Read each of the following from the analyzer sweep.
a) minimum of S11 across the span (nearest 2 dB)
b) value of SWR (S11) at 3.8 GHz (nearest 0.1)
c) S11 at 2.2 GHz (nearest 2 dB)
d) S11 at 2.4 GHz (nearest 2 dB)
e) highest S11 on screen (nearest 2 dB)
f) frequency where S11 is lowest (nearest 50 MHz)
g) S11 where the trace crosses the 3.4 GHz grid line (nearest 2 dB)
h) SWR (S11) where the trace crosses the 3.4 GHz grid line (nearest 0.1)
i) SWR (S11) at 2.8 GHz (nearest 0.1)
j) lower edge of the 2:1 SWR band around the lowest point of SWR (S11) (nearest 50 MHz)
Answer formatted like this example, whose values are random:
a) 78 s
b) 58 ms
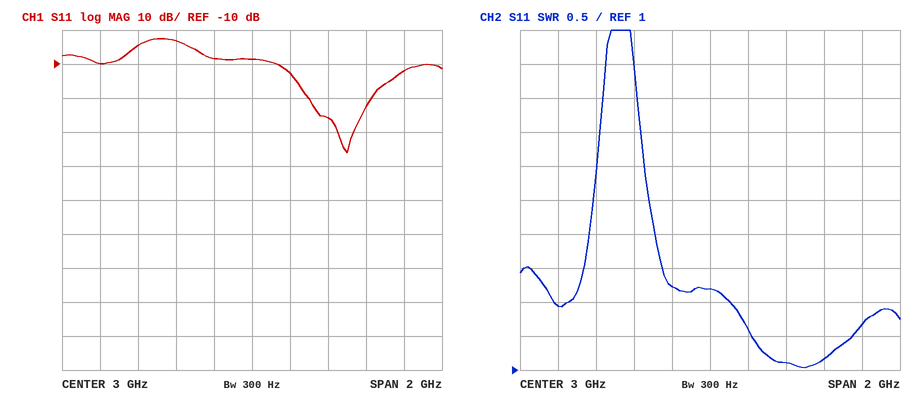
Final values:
a) -36 dB
b) 1.7
c) -10 dB
d) -4 dB
e) -2 dB
f) 3.50 GHz
g) -26 dB
h) 1.1
i) 2.2
j) 3.10 GHz
